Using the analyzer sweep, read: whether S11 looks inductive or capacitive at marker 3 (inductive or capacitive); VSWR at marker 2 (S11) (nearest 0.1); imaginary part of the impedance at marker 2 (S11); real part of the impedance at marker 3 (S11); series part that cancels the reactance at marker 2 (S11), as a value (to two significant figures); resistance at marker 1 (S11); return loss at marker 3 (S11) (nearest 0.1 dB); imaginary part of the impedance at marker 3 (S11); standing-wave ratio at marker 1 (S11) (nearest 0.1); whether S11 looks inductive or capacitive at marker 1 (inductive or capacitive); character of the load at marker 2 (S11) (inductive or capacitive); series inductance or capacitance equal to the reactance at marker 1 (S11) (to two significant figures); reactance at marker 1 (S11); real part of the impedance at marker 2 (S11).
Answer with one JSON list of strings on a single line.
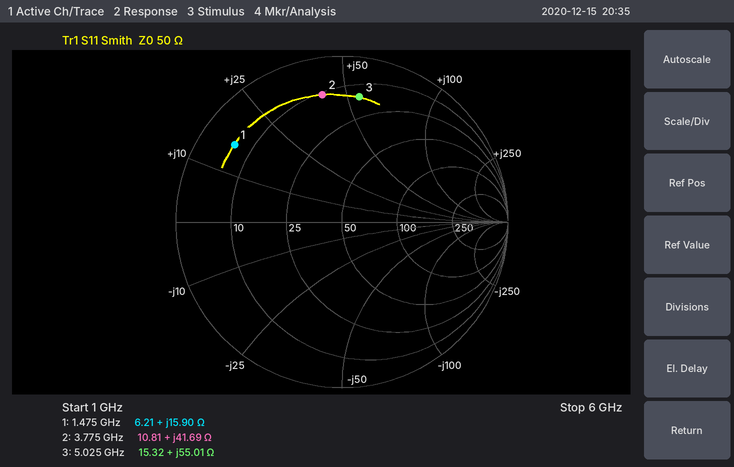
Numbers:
["inductive", "7.9", "+41.69 Ω", "15.32 Ω", "1.0 pF", "6.21 Ω", "2.4 dB", "+55.01 Ω", "8.9", "inductive", "inductive", "1.7 nH", "+15.90 Ω", "10.81 Ω"]
